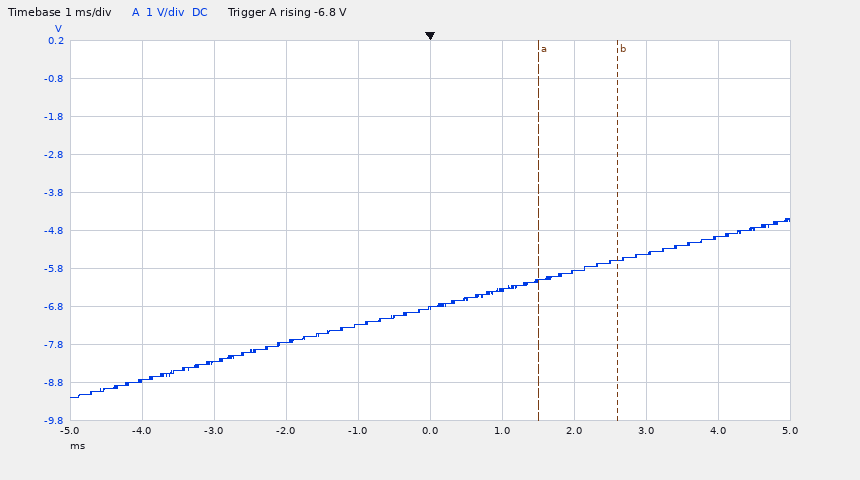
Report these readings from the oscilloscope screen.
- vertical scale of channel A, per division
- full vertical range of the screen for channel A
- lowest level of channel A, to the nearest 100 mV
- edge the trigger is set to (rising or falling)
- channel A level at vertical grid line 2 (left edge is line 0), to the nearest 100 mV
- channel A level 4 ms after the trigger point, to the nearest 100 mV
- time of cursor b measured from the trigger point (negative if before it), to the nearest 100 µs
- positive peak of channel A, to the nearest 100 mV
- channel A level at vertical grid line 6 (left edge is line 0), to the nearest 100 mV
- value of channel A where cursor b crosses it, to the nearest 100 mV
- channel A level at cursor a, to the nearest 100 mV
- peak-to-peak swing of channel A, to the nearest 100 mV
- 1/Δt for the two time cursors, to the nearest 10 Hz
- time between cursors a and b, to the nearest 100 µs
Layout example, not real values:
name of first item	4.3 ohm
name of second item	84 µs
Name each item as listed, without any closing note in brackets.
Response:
vertical scale of channel A, per division	1 V
full vertical range of the screen for channel A	10 V
lowest level of channel A, to the nearest 100 mV	-9.2 V
edge the trigger is set to	rising
channel A level at vertical grid line 2 (left edge is line 0), to the nearest 100 mV	-8.3 V
channel A level 4 ms after the trigger point, to the nearest 100 mV	-5.0 V
time of cursor b measured from the trigger point (negative if before it), to the nearest 100 µs	+2.6 ms
positive peak of channel A, to the nearest 100 mV	-4.5 V
channel A level at vertical grid line 6 (left edge is line 0), to the nearest 100 mV	-6.4 V
value of channel A where cursor b crosses it, to the nearest 100 mV	-5.6 V
channel A level at cursor a, to the nearest 100 mV	-6.1 V
peak-to-peak swing of channel A, to the nearest 100 mV	4.7 V
1/Δt for the two time cursors, to the nearest 10 Hz	910 Hz
time between cursors a and b, to the nearest 100 µs	1.1 ms
